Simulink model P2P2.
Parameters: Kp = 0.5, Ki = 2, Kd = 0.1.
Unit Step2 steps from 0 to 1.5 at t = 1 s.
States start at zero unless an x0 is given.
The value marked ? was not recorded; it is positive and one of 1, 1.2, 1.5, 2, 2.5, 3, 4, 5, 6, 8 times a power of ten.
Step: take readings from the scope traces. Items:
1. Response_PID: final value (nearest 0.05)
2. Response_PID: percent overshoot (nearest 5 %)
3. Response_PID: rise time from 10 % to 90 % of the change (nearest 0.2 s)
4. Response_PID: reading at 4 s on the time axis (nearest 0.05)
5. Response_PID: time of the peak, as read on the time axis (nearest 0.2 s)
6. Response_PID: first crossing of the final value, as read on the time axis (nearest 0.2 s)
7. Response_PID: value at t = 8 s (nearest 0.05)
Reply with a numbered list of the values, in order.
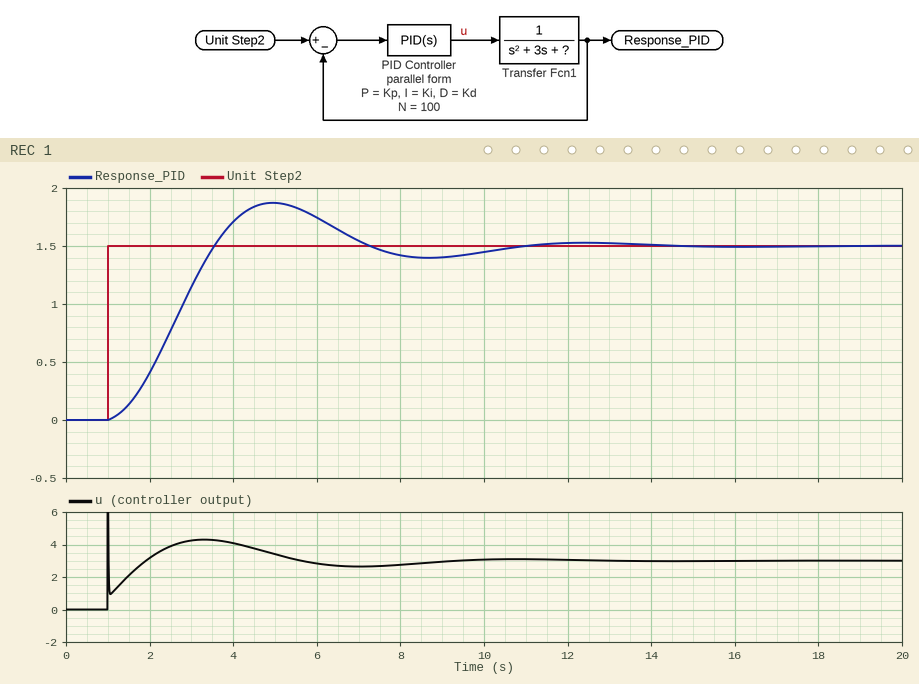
1. 1.50
2. 25 %
3. 1.8 s
4. 1.70
5. 5.0 s
6. 3.6 s
7. 1.40
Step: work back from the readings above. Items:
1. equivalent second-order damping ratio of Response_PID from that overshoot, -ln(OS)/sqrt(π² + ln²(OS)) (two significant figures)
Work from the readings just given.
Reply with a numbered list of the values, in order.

1. 0.40
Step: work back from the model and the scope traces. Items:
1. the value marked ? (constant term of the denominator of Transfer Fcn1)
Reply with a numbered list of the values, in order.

1. 2
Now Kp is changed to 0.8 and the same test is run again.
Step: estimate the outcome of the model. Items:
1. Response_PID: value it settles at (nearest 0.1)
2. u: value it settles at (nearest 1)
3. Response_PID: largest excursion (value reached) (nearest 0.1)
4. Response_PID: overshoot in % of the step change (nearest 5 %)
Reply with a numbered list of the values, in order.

1. 1.5
2. 3
3. 1.8
4. 20 %
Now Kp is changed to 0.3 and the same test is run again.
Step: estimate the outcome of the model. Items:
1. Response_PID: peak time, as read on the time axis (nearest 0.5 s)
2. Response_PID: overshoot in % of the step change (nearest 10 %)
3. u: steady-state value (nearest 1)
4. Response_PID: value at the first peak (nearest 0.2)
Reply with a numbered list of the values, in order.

1. 5.0 s
2. 30 %
3. 3
4. 2.0
